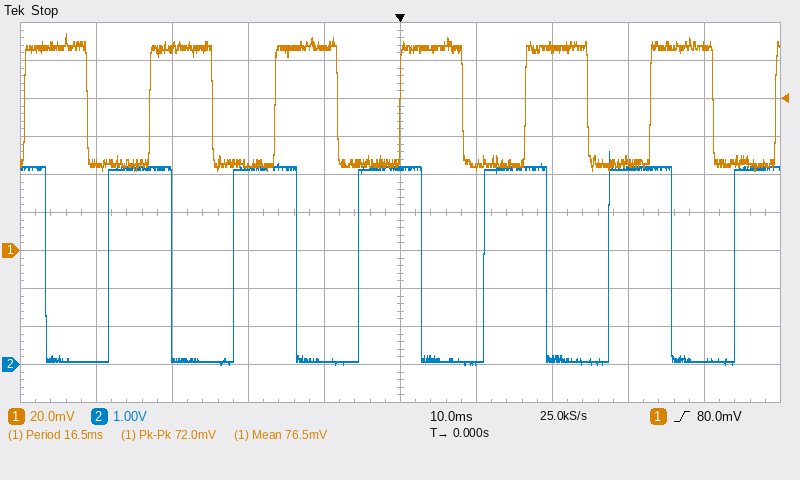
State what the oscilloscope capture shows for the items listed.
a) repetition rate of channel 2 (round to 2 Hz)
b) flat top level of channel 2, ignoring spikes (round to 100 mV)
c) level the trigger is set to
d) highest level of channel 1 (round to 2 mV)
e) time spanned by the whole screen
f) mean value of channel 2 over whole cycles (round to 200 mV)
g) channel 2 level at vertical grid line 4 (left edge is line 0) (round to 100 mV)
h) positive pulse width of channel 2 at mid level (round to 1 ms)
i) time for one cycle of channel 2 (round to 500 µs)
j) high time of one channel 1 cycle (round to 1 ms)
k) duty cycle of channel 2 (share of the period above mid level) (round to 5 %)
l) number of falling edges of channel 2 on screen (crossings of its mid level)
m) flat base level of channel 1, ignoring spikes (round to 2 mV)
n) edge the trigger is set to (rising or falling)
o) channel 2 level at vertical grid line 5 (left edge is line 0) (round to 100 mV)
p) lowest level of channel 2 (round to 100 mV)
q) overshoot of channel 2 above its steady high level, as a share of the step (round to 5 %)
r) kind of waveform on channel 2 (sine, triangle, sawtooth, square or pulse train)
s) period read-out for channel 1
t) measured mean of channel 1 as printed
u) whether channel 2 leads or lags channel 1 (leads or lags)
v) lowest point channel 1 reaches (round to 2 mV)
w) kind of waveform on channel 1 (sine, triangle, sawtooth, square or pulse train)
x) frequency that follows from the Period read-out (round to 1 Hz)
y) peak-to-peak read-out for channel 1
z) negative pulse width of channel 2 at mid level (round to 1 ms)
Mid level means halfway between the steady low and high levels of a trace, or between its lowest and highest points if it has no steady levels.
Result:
60 Hz
5.2 V
80.0 mV
114 mV
100 ms
2.6 V
100 mV
8 ms
16.5 ms
8 ms
50 %
6
46 mV
rising
5.2 V
0.0 V
10 %
square
16.5 ms
76.5 mV
leads
42 mV
square
61 Hz
72.0 mV
8 ms
